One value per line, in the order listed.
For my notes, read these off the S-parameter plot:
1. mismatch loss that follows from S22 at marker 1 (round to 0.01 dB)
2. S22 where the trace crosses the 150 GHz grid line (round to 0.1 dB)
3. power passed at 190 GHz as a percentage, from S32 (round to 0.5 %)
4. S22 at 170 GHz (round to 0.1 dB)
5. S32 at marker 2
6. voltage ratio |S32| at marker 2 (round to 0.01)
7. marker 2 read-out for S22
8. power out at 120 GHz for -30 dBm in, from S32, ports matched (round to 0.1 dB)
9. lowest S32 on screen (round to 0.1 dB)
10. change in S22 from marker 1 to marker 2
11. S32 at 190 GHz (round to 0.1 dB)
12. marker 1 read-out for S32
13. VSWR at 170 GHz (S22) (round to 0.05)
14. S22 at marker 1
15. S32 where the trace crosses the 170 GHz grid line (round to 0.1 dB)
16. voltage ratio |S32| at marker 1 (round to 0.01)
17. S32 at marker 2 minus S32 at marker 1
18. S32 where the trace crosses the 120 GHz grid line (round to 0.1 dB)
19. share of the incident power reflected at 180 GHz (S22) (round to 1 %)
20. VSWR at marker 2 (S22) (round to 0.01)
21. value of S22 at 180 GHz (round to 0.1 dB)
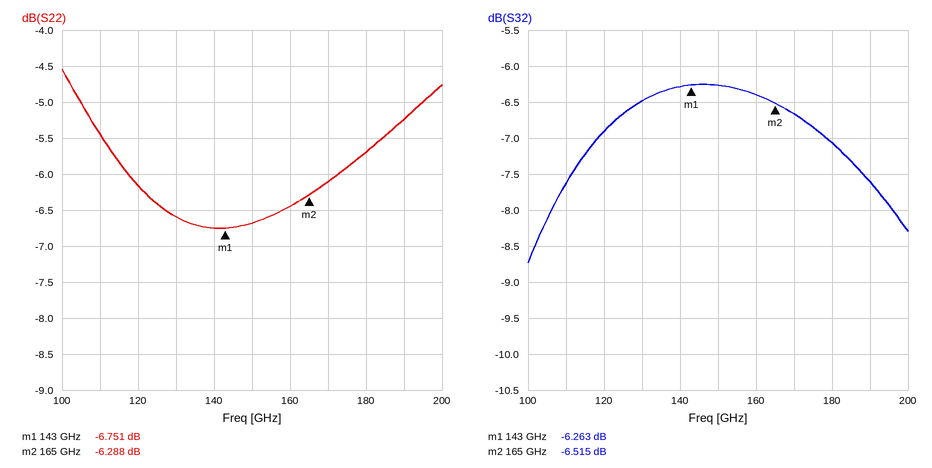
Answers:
1.03 dB
-6.7 dB
17.5 %
-6.1 dB
-6.515 dB
0.47
-6.288 dB
-36.9 dBm
-8.7 dB
0.463 dB
-7.6 dB
-6.263 dB
2.95
-6.751 dB
-6.7 dB
0.49
-0.252 dB
-6.9 dB
27 %
2.88
-5.7 dB
